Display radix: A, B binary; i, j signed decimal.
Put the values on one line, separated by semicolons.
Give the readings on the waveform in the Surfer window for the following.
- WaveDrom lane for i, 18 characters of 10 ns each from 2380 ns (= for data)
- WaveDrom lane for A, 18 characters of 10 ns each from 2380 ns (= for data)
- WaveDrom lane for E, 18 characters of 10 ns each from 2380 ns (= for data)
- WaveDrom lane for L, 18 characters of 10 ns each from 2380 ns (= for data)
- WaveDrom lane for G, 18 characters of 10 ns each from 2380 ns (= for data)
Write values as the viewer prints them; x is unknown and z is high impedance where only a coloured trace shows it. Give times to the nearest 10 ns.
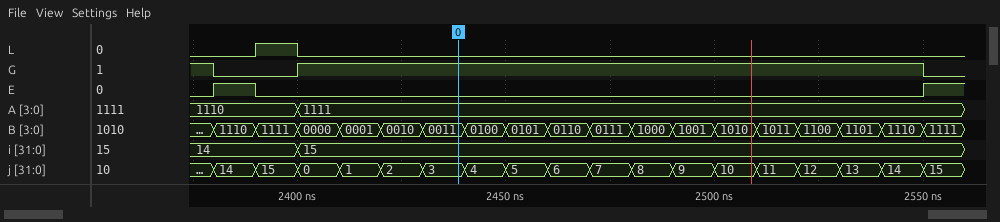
{name: 'i', wave: '=.=...............', data: '14 15'}; {name: 'A', wave: '=.=...............', data: '1110 1111'}; {name: 'E', wave: '10...............1'}; {name: 'L', wave: '010...............'}; {name: 'G', wave: '0.1..............0'}
